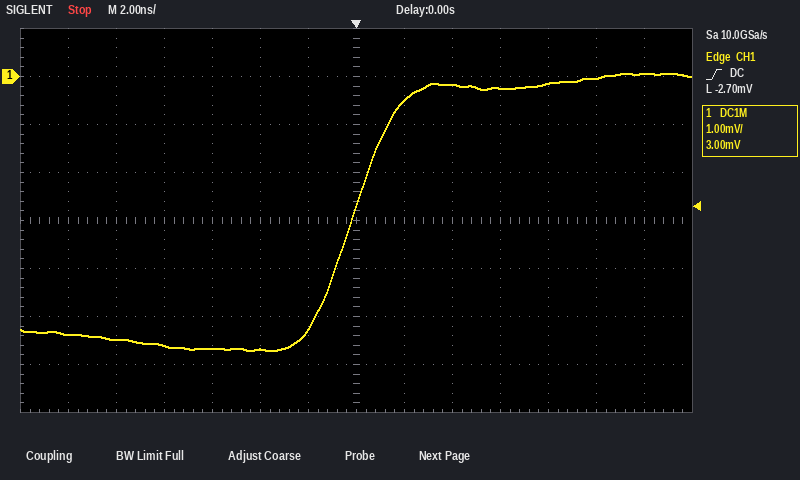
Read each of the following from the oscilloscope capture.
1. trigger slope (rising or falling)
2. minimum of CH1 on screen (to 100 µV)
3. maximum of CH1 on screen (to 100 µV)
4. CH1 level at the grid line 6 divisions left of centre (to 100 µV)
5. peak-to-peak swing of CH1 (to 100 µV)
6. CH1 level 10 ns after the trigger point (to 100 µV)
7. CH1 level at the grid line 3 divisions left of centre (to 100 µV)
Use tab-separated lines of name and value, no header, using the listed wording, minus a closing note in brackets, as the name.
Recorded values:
trigger slope	rising
minimum of CH1 on screen	-5.7 mV
maximum of CH1 on screen	100 µV
CH1 level at the grid line 6 divisions left of centre	-5.4 mV
peak-to-peak swing of CH1	5.8 mV
CH1 level 10 ns after the trigger point	0.0 mV
CH1 level at the grid line 3 divisions left of centre	-5.7 mV
